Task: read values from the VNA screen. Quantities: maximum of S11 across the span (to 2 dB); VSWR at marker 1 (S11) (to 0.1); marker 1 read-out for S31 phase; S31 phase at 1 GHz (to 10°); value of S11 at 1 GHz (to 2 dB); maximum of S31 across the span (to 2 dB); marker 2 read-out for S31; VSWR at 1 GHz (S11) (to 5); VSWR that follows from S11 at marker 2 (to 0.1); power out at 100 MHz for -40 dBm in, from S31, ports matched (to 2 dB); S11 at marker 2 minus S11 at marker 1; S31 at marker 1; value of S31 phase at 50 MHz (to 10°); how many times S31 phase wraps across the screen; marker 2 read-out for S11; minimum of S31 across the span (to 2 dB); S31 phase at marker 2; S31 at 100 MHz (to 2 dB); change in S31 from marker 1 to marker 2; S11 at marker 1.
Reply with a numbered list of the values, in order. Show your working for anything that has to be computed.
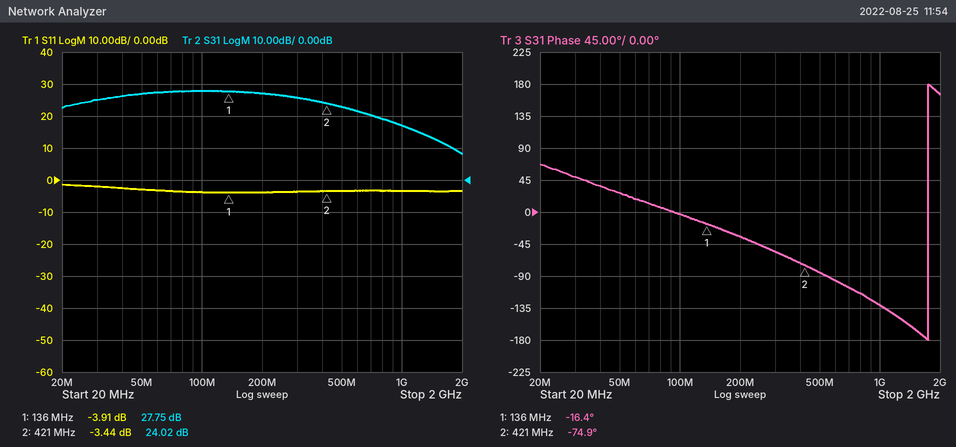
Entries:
1. -2 dB
2. (1 + 0.6375)/(1 − 0.6375) ≈ 4.5
3. -16.4°
4. -130°
5. -4 dB
6. 28 dB
7. 24.02 dB
8. |Γ| = 10^(-4/20) = 0.6310; VSWR = (1 + 0.6310)/(1 − 0.6310) ≈ 4.42, so 5 to the nearest 5
9. (1 + 0.6730)/(1 − 0.6730) ≈ 5.1
10. -40 dBm + (28 dB) = -12 dBm
11. -3.44 − (-3.91) = 0.47 dB
12. 27.75 dB
13. 30°
14. 1
15. -3.44 dB
16. 8 dB
17. -74.9°
18. 28 dB
19. 24.02 − (27.75) = -3.73 dB
20. -3.91 dB
